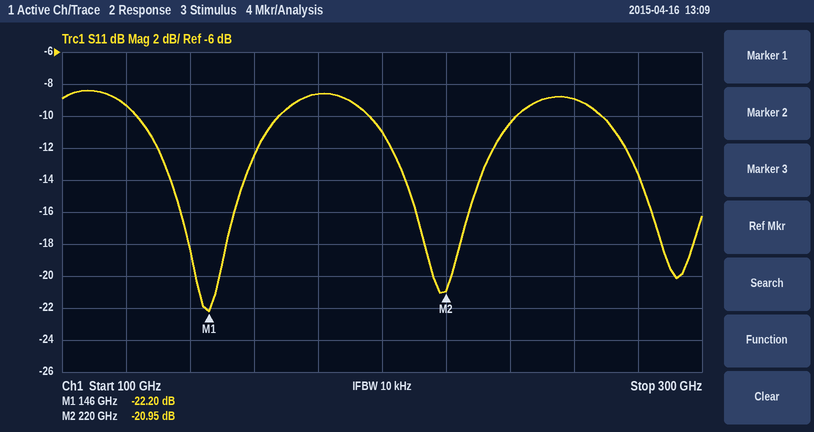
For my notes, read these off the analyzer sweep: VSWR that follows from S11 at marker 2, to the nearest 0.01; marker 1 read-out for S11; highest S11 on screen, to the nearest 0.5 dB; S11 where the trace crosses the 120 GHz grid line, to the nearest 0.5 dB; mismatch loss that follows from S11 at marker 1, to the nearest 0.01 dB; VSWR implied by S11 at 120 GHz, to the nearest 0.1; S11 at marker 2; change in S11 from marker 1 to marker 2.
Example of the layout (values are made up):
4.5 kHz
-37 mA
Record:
1.20
-22.20 dB
-8.5 dB
-9.5 dB
0.03 dB
2.0
-20.95 dB
1.25 dB
